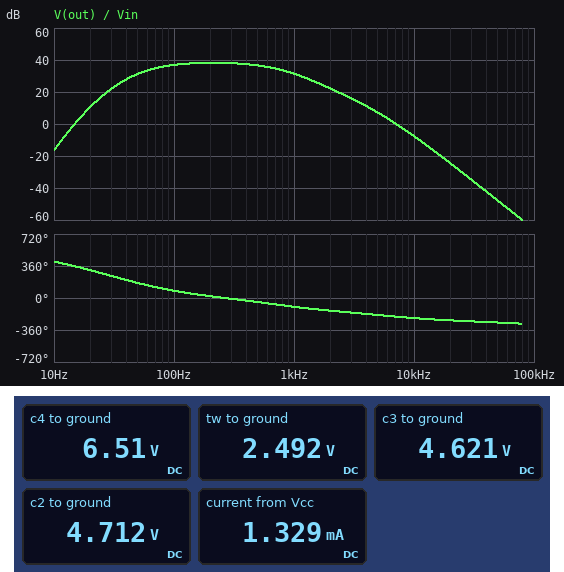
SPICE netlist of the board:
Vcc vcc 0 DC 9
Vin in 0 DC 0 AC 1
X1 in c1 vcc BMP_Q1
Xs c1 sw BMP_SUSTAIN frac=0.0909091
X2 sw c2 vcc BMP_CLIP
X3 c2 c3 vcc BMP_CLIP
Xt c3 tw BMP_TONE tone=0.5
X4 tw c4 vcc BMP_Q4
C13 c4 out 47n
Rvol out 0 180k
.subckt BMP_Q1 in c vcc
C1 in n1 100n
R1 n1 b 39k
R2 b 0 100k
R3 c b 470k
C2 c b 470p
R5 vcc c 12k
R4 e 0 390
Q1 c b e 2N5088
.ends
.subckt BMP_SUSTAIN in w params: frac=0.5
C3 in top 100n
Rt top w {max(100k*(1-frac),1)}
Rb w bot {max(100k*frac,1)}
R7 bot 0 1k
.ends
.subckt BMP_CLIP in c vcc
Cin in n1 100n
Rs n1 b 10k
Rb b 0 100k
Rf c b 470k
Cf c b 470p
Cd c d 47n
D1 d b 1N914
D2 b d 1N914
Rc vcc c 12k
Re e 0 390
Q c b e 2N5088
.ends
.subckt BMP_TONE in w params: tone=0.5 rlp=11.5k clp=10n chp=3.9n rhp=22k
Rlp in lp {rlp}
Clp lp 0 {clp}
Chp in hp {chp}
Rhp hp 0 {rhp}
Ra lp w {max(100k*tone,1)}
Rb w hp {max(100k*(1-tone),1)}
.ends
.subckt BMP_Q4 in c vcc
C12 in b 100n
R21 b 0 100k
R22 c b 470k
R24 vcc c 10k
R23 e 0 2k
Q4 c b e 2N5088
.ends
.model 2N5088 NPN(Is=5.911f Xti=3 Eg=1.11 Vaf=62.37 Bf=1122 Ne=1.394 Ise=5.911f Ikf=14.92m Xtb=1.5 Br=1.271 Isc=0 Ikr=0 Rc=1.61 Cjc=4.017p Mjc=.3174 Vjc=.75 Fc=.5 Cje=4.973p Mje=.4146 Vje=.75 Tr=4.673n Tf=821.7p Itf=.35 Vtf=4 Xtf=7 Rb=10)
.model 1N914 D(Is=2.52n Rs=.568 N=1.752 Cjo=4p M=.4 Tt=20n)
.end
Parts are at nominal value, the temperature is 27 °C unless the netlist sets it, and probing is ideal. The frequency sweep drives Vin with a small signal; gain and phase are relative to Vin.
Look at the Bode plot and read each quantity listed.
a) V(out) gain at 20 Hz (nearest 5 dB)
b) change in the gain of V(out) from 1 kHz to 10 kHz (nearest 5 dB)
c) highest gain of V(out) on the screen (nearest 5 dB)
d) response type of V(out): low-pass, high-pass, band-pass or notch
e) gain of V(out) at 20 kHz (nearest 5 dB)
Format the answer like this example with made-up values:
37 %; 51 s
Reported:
10 dB; -40 dB; 40 dB; band-pass; -25 dB
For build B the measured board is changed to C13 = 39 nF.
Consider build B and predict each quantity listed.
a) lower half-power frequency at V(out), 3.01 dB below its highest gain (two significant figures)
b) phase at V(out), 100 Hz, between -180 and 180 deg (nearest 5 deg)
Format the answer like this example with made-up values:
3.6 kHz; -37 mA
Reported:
75 Hz; 85 deg
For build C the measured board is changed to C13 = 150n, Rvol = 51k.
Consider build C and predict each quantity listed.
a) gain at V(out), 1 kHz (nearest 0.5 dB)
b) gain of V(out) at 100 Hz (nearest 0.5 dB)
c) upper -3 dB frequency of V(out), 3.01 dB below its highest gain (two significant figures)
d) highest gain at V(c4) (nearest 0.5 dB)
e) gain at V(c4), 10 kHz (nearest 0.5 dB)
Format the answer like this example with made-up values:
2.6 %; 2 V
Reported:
30.5 dB; 36.0 dB; 640 Hz; 37.5 dB; -8.5 dB
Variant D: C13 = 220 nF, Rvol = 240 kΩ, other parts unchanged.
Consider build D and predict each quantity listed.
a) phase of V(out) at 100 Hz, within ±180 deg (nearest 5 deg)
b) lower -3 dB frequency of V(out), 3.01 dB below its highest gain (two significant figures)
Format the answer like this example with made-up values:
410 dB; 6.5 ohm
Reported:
75 deg; 72 Hz
